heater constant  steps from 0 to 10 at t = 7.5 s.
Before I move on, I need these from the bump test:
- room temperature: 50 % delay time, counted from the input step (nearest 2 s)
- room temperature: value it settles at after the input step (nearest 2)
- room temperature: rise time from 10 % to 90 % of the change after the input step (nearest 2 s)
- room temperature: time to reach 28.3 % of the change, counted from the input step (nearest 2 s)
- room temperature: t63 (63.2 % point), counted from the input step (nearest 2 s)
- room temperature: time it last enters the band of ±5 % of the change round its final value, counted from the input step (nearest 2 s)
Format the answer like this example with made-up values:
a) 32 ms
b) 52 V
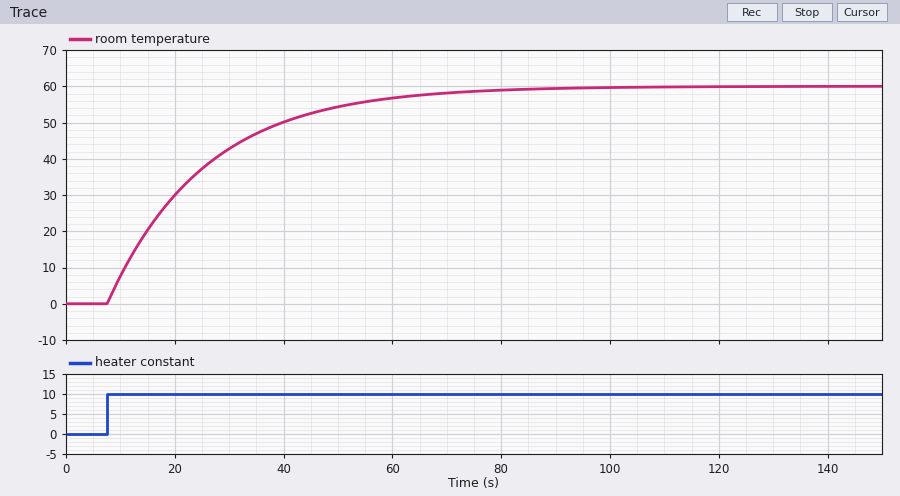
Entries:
a) 12 s
b) 60
c) 40 s
d) 6 s
e) 18 s
f) 54 s
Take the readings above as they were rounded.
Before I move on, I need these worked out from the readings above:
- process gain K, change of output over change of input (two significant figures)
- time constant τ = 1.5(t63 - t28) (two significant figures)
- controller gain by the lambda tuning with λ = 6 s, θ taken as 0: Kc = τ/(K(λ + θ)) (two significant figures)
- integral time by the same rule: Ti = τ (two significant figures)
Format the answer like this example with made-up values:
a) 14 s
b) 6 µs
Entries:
a) 6.0
b) 18 s
c) 0.50
d) 18 s
